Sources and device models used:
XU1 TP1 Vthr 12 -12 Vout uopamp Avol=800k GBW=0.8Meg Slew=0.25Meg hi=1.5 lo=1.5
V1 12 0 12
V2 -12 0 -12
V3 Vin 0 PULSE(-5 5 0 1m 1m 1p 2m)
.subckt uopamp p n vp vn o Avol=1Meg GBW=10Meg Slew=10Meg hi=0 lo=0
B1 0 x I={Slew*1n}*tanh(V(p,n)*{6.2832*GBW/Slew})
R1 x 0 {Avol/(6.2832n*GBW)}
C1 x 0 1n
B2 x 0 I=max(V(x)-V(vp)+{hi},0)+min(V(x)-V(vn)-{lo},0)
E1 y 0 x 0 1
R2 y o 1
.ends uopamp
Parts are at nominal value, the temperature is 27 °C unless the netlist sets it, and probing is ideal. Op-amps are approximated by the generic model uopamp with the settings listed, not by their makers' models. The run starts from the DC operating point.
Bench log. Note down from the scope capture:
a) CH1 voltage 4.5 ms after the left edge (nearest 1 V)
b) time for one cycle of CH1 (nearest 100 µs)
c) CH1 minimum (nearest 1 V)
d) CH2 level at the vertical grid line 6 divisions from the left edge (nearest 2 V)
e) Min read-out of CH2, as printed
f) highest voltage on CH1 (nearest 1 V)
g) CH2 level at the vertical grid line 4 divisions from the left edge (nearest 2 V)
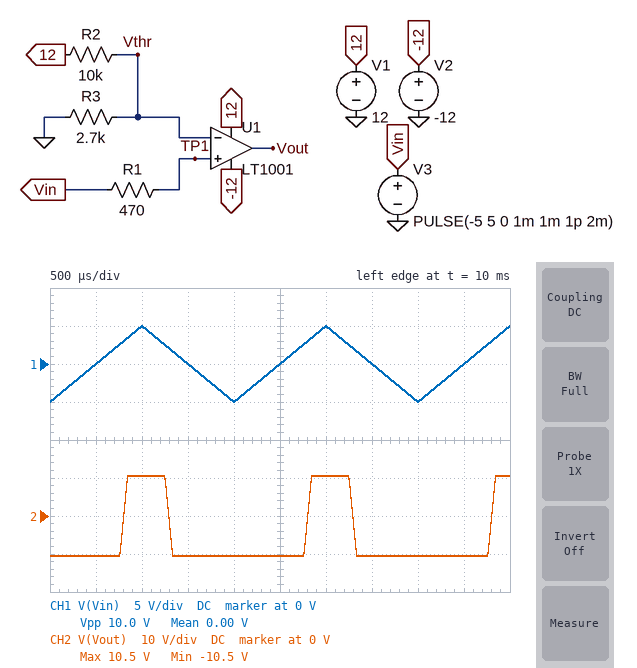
0 V
2.0 ms
-5 V
10 V
-10.5 V
5 V
-10 V
